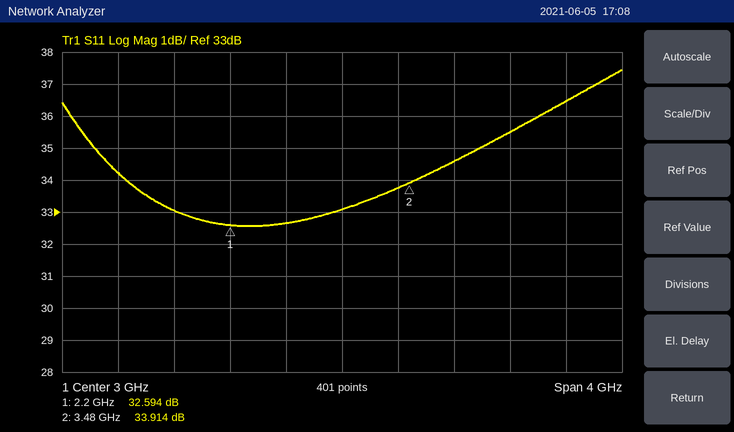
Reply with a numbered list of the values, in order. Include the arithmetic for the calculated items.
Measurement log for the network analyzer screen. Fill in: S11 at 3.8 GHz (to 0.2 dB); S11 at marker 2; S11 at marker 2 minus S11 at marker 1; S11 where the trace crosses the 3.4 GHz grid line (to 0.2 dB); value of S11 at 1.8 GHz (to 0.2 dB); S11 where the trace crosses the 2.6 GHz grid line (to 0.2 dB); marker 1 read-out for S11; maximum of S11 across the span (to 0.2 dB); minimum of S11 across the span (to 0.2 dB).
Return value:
1. 34.6 dB
2. 33.914 dB
3. 33.914 − (32.594) = 1.320 dB
4. 33.8 dB
5. 33.0 dB
6. 32.6 dB
7. 32.594 dB
8. 37.4 dB
9. 32.6 dB
